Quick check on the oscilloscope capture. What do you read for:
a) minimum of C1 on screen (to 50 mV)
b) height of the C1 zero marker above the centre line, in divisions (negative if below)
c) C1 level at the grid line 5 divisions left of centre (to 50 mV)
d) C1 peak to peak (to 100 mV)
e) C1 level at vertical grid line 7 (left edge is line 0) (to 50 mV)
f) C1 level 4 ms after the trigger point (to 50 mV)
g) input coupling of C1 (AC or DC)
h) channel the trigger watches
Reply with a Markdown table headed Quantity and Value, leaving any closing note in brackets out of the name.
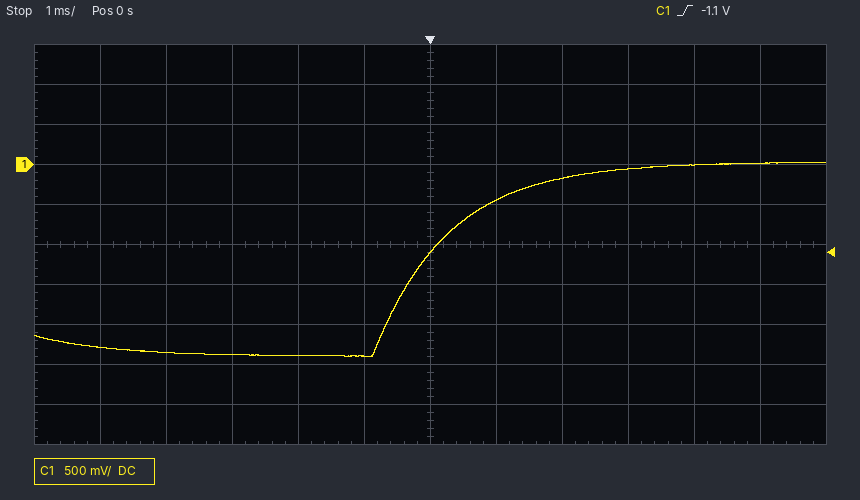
| Quantity | Value |
|---|---|
| minimum of C1 on screen | -2.40 V |
| height of the C1 zero marker above the centre line, in divisions | +2.0 div |
| C1 level at the grid line 5 divisions left of centre | -2.30 V |
| C1 peak to peak | 2.40 V |
| C1 level at vertical grid line 7 (left edge is line 0) | -450 mV |
| C1 level 4 ms after the trigger point | 0 mV |
| input coupling of C1 | DC |
| channel the trigger watches | C1 |
